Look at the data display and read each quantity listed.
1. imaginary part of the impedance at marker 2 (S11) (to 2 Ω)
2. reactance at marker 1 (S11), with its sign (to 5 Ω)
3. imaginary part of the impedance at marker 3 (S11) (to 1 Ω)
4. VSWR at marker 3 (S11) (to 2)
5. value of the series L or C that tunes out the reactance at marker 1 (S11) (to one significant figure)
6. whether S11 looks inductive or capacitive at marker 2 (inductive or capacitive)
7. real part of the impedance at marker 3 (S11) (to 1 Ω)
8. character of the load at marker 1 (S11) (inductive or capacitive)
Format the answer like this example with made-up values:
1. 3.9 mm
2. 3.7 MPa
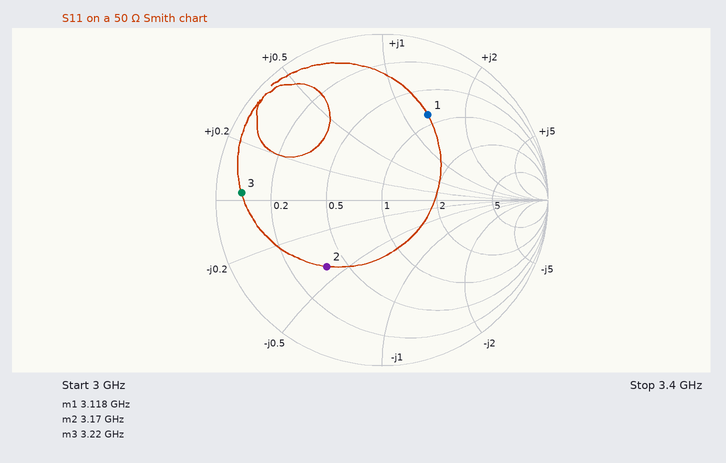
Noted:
1. -20 Ω
2. +65 Ω
3. +1 Ω
4. 12
5. 800 fF
6. capacitive
7. 4 Ω
8. inductive
